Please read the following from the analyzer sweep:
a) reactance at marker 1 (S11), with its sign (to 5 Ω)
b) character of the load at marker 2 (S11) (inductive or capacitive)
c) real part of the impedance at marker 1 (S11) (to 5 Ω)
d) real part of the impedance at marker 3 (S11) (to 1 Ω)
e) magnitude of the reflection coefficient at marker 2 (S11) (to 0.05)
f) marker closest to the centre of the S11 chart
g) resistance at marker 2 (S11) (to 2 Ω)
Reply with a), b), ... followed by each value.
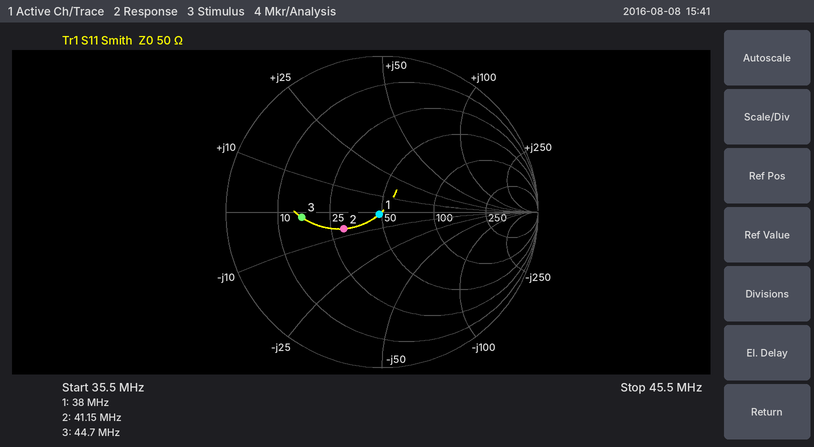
a) 0 Ω
b) capacitive
c) 50 Ω
d) 16 Ω
e) 0.25
f) marker 1
g) 30 Ω
